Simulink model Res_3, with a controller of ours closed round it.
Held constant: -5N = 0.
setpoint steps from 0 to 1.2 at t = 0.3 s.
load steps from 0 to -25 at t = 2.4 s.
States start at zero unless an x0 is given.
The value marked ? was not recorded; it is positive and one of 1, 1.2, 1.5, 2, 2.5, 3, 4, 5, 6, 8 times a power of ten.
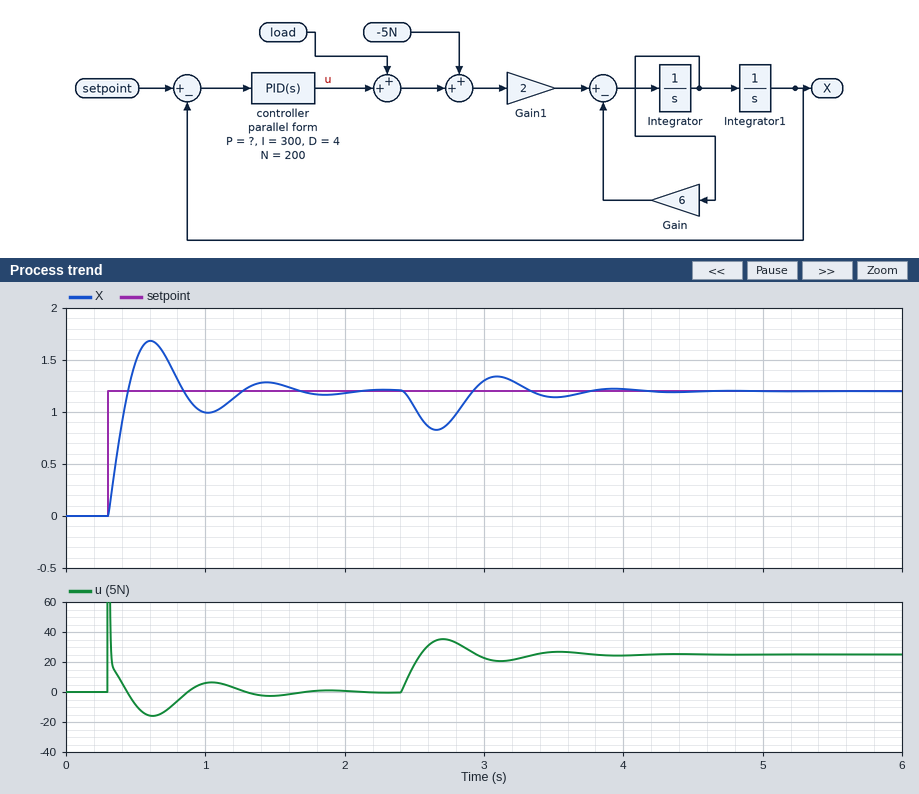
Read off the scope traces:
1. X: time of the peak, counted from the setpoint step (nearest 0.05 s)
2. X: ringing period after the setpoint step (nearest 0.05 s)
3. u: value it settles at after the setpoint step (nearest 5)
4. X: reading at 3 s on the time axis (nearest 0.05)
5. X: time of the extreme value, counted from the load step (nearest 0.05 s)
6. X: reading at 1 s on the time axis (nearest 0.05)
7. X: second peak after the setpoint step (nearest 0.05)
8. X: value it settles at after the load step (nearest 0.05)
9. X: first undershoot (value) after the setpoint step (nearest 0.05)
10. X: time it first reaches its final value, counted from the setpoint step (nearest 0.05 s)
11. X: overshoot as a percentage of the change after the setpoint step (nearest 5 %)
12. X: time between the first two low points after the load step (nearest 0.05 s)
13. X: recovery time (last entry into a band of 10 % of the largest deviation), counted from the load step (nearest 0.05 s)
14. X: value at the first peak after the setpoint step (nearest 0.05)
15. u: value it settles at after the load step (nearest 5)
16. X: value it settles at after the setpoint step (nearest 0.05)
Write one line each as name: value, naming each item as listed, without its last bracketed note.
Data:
X: time of the peak, counted from the setpoint step: 0.30 s
X: ringing period after the setpoint step: 0.85 s
u: value it settles at after the setpoint step: 0
X: reading at 3 s on the time axis: 1.30
X: time of the extreme value, counted from the load step: 0.25 s
X: reading at 1 s on the time axis: 1.00
X: second peak after the setpoint step: 1.30
X: value it settles at after the load step: 1.20
X: first undershoot (value) after the setpoint step: 1.00
X: time it first reaches its final value, counted from the setpoint step: 0.15 s
X: overshoot as a percentage of the change after the setpoint step: 40 %
X: time between the first two low points after the load step: 0.85 s
X: recovery time (last entry into a band of 10 % of the largest deviation), counted from the load step: 1.25 s
X: value at the first peak after the setpoint step: 1.70
u: value it settles at after the load step: 25
X: value it settles at after the setpoint step: 1.20
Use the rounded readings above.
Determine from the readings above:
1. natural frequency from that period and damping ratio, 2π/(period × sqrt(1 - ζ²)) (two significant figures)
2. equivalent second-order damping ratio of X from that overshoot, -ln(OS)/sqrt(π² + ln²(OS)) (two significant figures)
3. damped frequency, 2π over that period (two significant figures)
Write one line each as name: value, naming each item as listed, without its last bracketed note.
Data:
natural frequency from that period and damping ratio, 2π/(period × sqrt(1 - ζ²)): 7.7 rad/s
equivalent second-order damping ratio of X from that overshoot, -ln(OS)/sqrt(π² + ln²(OS)): 0.28
damped frequency, 2π over that period: 7.4 rad/s
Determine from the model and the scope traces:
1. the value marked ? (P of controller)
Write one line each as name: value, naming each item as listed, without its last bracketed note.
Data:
the value marked ?: 50
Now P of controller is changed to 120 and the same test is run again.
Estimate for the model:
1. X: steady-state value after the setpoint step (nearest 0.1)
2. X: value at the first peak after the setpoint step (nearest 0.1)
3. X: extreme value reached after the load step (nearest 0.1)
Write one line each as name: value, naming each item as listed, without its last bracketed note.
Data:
X: steady-state value after the setpoint step: 1.2
X: value at the first peak after the setpoint step: 1.6
X: extreme value reached after the load step: 1.0
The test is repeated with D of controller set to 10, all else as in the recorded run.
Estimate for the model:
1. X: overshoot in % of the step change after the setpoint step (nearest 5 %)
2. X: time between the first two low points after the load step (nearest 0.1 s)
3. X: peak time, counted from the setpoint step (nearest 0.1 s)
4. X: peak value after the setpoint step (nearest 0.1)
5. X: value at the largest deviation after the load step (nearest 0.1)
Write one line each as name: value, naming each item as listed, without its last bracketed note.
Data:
X: overshoot in % of the step change after the setpoint step: 15 %
X: time between the first two low points after the load step: 1.3 s
X: peak time, counted from the setpoint step: 0.4 s
X: peak value after the setpoint step: 1.4
X: value at the largest deviation after the load step: 0.9
